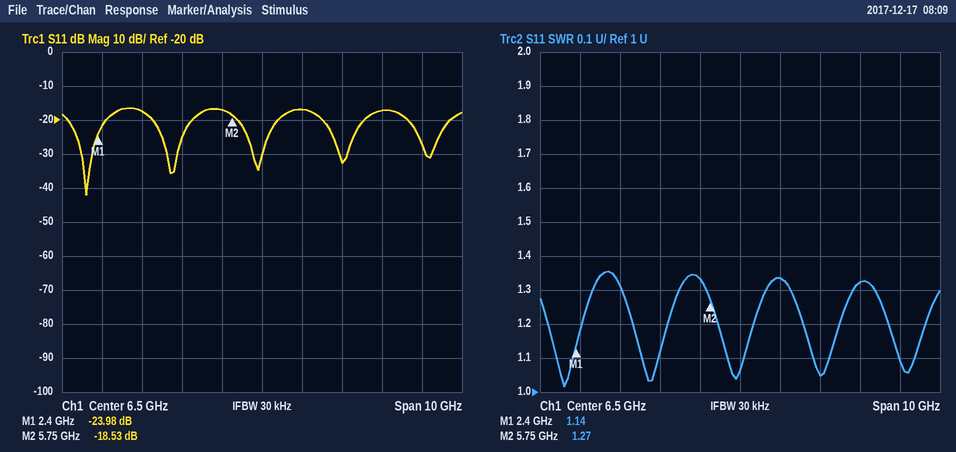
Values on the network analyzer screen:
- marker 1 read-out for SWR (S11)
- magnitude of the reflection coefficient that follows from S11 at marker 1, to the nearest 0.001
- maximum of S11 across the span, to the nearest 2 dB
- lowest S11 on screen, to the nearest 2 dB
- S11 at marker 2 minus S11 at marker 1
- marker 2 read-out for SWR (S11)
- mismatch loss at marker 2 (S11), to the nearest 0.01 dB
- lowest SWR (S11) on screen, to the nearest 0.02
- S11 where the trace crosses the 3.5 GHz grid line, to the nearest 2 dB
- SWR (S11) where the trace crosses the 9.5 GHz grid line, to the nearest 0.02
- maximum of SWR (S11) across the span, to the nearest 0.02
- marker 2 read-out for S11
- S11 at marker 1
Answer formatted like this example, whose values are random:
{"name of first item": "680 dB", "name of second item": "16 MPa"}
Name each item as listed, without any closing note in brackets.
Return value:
{"marker 1 read-out for SWR": "1.14", "magnitude of the reflection coefficient that follows from S11 at marker 1, to the nearest 0.001": "0.063", "maximum of S11 across the span, to the nearest 2 dB": "-16 dB", "lowest S11 on screen, to the nearest 2 dB": "-42 dB", "S11 at marker 2 minus S11 at marker 1": "5.45 dB", "marker 2 read-out for SWR": "1.27", "mismatch loss at marker 2 (S11), to the nearest 0.01 dB": "0.06 dB", "lowest SWR (S11) on screen, to the nearest 0.02": "1.02", "S11 where the trace crosses the 3.5 GHz grid line, to the nearest 2 dB": "-18 dB", "SWR (S11) where the trace crosses the 9.5 GHz grid line, to the nearest 0.02": "1.32", "maximum of SWR (S11) across the span, to the nearest 0.02": "1.36", "marker 2 read-out for S11": "-18.53 dB", "S11 at marker 1": "-23.98 dB"}
